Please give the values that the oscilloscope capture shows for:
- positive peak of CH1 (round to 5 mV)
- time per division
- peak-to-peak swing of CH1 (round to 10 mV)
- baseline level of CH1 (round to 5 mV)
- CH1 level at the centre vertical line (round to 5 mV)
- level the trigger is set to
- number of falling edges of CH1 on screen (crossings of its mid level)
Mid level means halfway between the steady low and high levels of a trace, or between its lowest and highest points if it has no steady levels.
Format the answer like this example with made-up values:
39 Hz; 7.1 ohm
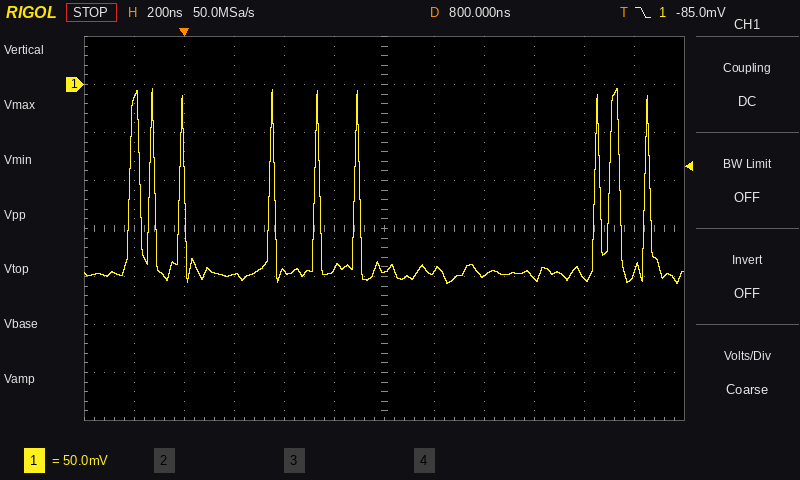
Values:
-5 mV; 200 ns; 200 mV; -195 mV; -195 mV; -85.0 mV; 9
